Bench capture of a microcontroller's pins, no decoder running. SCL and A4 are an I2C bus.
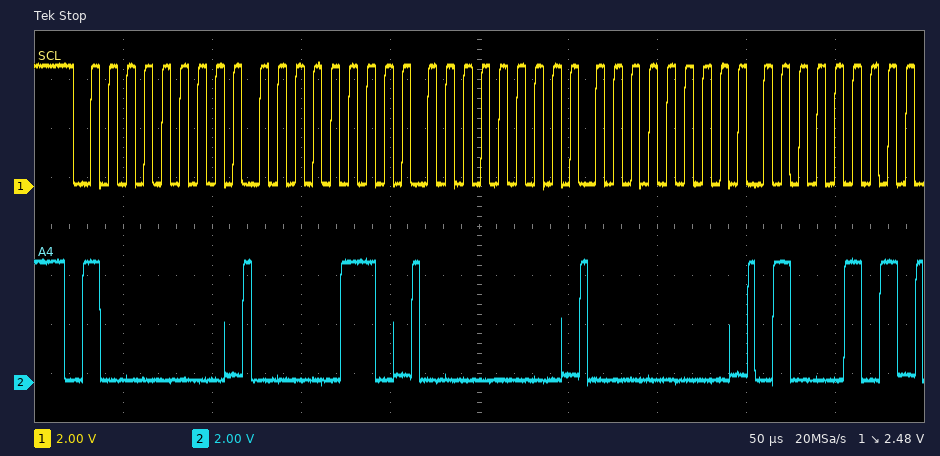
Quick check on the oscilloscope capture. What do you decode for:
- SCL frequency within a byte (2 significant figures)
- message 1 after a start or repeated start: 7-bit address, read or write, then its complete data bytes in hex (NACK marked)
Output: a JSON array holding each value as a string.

["100 kHz", "0x40 write: 06 00 00 45"]
